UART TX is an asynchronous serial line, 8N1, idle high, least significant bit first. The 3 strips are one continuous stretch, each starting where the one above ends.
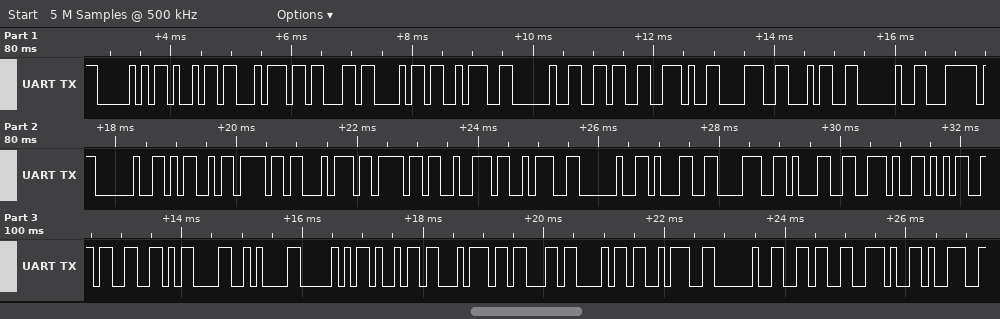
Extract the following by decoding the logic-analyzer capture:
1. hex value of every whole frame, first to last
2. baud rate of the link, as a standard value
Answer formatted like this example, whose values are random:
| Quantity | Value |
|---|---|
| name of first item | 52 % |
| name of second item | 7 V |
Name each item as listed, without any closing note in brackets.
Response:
| Quantity | Value |
|---|---|
| hex value of every whole frame, first to last | 50 69 74 63 68 3A 20 36 2E 38 34 20 7C 20 4D 6F 74 6F 72 3A 20 31 38 31 2E 35 33 0D 0A 50 69 74 63 68 3A 20 36 2E 39 |
| baud rate of the link, as a standard value | 9600 baud |
